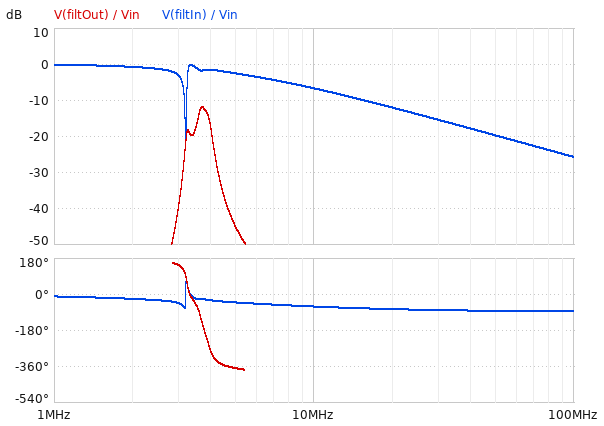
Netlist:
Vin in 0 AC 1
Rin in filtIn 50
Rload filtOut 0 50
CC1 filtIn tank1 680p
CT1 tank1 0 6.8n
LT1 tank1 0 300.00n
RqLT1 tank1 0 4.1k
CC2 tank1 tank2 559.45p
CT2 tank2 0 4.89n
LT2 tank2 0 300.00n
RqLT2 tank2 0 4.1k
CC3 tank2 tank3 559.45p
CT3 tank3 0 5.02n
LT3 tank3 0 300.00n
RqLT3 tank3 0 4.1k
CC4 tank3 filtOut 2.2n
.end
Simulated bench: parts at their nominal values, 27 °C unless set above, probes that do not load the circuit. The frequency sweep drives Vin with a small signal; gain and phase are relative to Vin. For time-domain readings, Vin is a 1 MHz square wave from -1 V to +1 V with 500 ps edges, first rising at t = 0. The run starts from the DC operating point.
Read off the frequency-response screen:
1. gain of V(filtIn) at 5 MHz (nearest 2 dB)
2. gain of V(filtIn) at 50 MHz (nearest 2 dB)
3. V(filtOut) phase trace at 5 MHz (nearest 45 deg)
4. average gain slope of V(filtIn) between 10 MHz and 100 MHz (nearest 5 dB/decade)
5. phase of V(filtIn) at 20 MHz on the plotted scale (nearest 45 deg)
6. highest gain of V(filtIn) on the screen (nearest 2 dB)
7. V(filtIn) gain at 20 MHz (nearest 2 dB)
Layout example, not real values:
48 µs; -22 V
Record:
-2 dB; -20 dB; -360 deg; -20 dB/decade; -90 deg; 0 dB; -12 dB
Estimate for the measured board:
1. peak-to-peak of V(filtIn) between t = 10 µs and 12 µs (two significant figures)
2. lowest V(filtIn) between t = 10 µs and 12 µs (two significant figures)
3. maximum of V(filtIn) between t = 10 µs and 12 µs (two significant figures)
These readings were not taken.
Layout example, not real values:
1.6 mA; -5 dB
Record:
2.2 V; -1.1 V; 1.1 V
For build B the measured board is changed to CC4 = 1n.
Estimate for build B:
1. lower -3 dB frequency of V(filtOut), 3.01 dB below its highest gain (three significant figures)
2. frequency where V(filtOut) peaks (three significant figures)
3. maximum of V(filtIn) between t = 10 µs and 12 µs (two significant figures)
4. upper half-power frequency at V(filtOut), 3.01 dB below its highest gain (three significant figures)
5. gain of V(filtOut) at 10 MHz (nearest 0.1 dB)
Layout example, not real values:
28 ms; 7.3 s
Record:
3.55 MHz; 3.64 MHz; 1.1 V; 3.98 MHz; -65.5 dB
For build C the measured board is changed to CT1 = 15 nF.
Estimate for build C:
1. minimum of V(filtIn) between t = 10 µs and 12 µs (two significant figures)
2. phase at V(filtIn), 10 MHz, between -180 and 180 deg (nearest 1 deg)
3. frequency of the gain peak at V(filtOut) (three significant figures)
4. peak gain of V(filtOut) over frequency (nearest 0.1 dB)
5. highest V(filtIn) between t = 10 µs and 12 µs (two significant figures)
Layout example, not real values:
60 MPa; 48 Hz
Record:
-1.0 V; -64 deg; 3.68 MHz; -25.6 dB; 1.0 V
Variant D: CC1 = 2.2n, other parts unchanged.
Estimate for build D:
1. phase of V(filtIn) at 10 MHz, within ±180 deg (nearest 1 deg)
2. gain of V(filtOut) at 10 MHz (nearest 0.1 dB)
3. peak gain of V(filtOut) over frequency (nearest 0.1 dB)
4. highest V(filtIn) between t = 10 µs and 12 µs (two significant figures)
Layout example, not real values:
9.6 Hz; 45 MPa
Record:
-79 deg; -64.2 dB; -9.1 dB; 1.1 V
